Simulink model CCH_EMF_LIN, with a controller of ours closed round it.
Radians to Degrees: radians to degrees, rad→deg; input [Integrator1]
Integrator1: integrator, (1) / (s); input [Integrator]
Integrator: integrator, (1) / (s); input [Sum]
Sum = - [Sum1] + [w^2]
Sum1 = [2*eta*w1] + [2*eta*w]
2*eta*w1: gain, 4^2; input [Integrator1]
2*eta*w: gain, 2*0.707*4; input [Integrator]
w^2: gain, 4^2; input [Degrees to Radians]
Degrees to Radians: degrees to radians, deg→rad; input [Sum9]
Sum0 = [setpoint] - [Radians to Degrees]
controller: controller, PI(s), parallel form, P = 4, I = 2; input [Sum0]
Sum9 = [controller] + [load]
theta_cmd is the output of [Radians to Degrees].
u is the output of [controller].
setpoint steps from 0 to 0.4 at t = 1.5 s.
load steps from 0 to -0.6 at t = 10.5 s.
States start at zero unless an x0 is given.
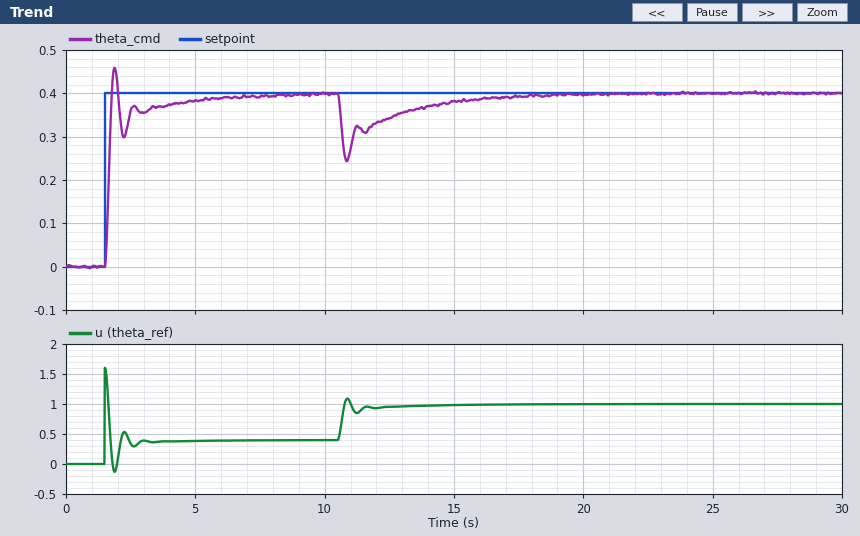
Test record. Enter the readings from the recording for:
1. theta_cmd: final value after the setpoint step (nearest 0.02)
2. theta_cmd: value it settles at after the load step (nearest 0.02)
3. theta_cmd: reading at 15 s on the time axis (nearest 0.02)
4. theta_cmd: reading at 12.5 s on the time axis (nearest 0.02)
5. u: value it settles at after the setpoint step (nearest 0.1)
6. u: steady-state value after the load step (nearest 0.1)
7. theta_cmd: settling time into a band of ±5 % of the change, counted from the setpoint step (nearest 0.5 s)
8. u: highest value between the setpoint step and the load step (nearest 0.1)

0.40
0.40
0.38
0.34
0.4
1.0
3.0 s
1.6
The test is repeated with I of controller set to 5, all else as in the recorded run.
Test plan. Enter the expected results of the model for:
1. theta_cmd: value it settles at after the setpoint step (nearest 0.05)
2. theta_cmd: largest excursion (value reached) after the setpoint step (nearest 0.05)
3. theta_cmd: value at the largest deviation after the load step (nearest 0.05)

0.40
0.50
0.25
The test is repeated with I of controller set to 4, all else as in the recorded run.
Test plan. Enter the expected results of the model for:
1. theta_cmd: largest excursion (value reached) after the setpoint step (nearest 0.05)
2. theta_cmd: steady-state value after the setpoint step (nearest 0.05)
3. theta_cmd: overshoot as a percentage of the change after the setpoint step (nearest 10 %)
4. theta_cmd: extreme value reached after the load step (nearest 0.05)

0.50
0.40
20 %
0.25
